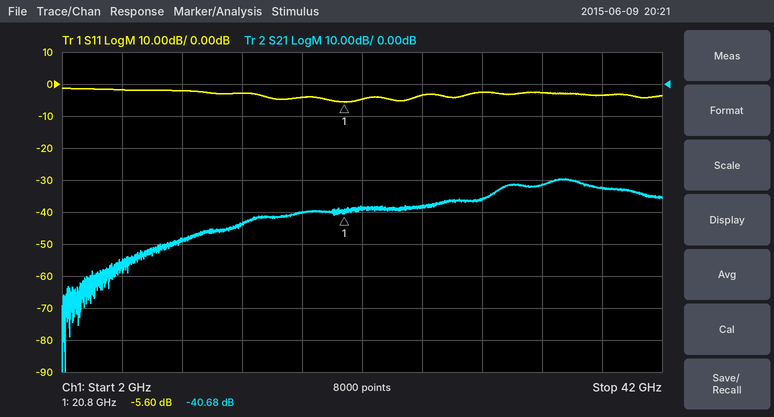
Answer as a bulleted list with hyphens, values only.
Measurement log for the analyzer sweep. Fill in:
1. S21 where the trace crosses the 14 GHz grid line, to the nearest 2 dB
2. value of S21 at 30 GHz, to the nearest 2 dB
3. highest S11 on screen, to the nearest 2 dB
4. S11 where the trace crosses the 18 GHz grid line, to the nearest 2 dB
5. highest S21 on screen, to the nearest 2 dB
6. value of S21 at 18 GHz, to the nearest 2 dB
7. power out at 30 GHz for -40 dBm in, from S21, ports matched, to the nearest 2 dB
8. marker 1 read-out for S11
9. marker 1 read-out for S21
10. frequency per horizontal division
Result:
- -44 dB
- -36 dB
- -2 dB
- -4 dB
- -30 dB
- -40 dB
- -76 dBm
- -5.60 dB
- -40.68 dB
- 4 GHz
